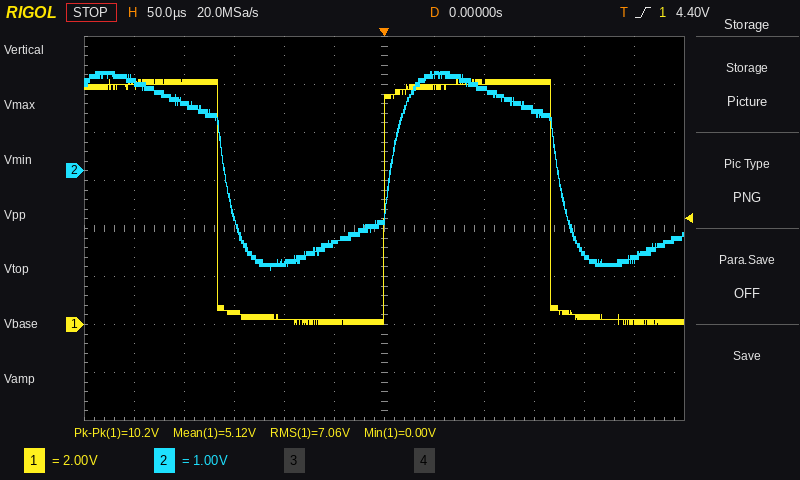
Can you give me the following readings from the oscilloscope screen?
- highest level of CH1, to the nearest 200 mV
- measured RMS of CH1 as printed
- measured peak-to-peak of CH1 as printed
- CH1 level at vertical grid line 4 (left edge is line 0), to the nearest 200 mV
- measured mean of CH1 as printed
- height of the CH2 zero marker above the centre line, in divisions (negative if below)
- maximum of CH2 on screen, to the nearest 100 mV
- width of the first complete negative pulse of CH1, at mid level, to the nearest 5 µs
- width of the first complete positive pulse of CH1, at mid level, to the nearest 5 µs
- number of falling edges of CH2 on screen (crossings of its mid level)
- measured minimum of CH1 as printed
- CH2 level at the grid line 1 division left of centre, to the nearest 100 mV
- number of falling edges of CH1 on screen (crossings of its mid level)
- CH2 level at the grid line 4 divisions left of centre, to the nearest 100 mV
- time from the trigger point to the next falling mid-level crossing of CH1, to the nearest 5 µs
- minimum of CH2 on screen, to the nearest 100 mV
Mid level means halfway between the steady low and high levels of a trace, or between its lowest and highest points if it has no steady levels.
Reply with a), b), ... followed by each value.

a) 10.2 V
b) 7.06 V
c) 10.2 V
d) 200 mV
e) 5.12 V
f) +1.2 div
g) 2.1 V
h) 165 µs
i) 165 µs
j) 2
k) 0.00 V
l) -1.5 V
m) 2
n) 1.4 V
o) 165 µs
p) -2.1 V
